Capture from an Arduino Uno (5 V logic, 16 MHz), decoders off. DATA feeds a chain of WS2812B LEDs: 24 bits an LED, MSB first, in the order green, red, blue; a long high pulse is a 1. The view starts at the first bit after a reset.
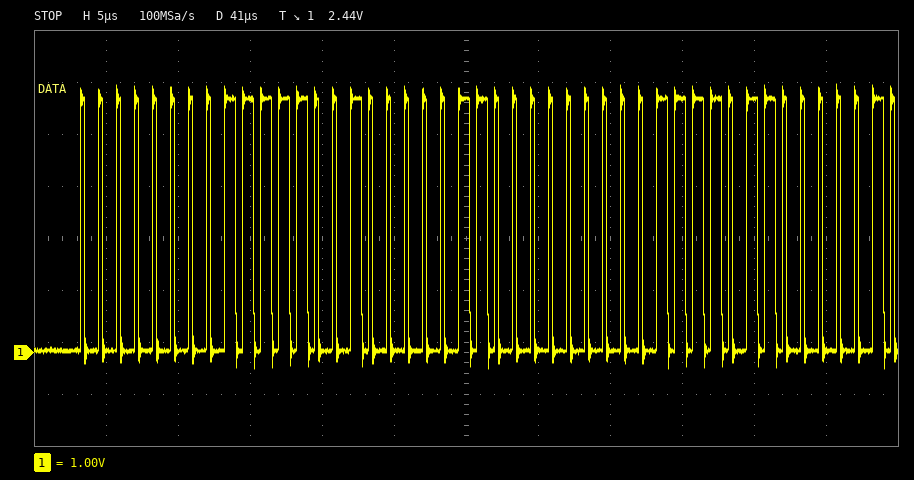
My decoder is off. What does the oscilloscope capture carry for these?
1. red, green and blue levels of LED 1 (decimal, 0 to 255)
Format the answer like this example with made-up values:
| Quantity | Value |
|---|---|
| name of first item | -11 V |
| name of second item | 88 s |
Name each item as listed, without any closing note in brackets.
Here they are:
| Quantity | Value |
|---|---|
| red, green and blue levels of LED 1 | 249, 0, 6 |
